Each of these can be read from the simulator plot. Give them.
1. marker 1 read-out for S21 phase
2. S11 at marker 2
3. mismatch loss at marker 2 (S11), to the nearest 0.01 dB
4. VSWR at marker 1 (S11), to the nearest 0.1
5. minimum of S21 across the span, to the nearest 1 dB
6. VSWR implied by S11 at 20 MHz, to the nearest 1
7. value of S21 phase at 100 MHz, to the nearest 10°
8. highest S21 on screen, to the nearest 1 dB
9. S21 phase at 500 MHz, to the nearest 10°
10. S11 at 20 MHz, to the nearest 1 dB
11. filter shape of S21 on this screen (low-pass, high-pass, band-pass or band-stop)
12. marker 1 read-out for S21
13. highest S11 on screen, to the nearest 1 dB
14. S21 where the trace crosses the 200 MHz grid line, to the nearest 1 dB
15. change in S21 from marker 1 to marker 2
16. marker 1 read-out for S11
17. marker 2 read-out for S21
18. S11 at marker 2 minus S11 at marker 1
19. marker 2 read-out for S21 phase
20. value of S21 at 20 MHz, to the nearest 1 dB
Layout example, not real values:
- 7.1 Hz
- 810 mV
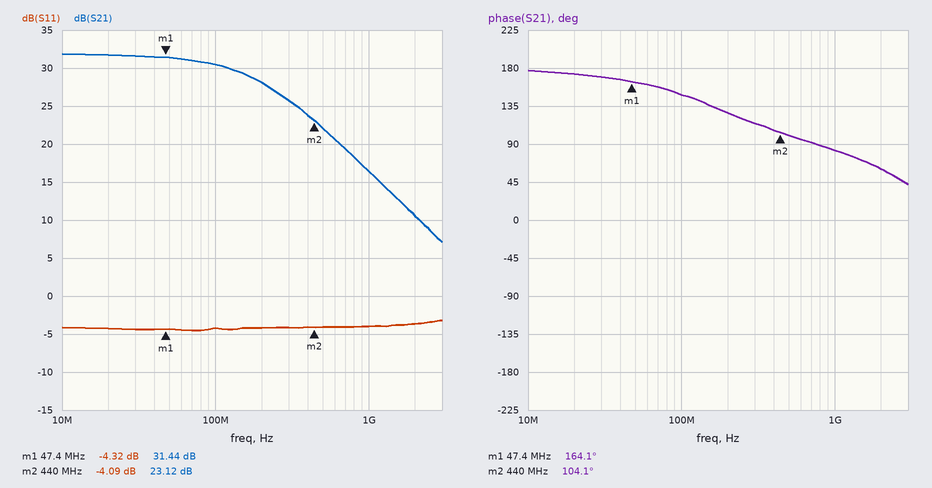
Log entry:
- 164.1°
- -4.09 dB
- 2.15 dB
- 4.1
- 7 dB
- 4
- 150°
- 32 dB
- 100°
- -4 dB
- low-pass
- 31.44 dB
- -3 dB
- 28 dB
- -8.32 dB
- -4.32 dB
- 23.12 dB
- 0.23 dB
- 104.1°
- 32 dB
